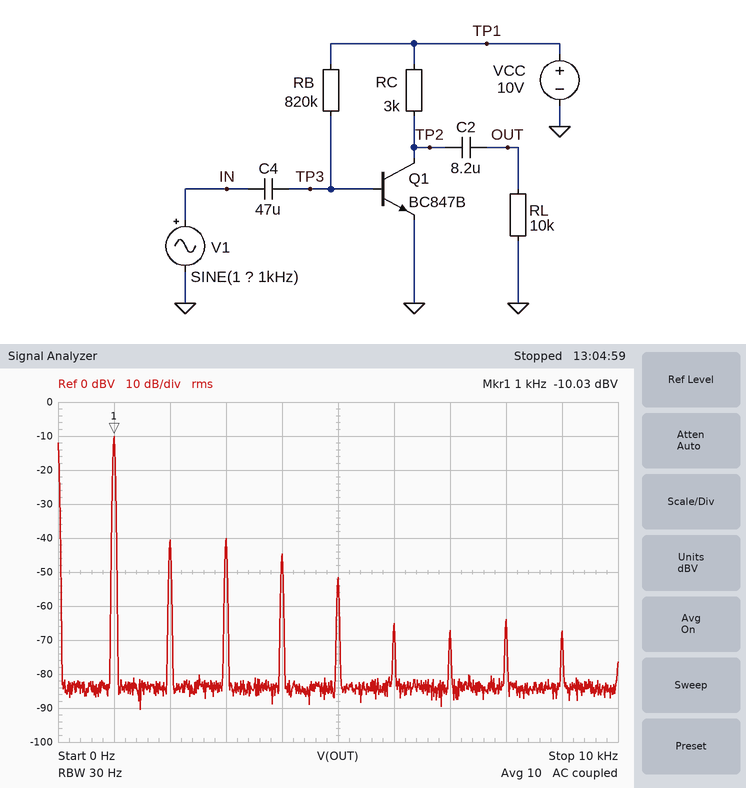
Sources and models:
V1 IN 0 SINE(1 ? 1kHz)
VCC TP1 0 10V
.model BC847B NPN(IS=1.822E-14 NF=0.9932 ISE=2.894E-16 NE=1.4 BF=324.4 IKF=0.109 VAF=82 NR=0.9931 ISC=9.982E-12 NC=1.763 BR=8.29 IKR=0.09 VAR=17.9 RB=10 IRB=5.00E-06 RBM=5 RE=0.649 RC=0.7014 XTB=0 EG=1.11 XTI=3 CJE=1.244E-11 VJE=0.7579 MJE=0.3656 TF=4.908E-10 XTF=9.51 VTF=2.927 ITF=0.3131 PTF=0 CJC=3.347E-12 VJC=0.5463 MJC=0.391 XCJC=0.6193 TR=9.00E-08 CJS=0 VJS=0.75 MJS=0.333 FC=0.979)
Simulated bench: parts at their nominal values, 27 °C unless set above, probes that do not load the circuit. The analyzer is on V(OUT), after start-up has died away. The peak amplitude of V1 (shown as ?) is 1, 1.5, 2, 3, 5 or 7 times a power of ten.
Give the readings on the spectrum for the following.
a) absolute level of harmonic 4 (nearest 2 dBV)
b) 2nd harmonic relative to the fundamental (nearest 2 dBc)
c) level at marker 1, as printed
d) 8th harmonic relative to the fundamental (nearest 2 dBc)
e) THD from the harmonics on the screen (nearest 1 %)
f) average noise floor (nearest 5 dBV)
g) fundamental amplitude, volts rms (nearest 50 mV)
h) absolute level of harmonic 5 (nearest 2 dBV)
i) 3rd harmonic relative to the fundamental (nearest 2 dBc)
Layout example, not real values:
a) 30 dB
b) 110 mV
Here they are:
a) -44 dBV
b) -30 dBc
c) -10.03 dBV
d) -54 dBc
e) 5 %
f) -85 dBV
g) 300 mV
h) -52 dBV
i) -30 dBc
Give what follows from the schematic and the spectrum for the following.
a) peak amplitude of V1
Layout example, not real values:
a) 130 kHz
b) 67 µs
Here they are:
a) 2 mV
